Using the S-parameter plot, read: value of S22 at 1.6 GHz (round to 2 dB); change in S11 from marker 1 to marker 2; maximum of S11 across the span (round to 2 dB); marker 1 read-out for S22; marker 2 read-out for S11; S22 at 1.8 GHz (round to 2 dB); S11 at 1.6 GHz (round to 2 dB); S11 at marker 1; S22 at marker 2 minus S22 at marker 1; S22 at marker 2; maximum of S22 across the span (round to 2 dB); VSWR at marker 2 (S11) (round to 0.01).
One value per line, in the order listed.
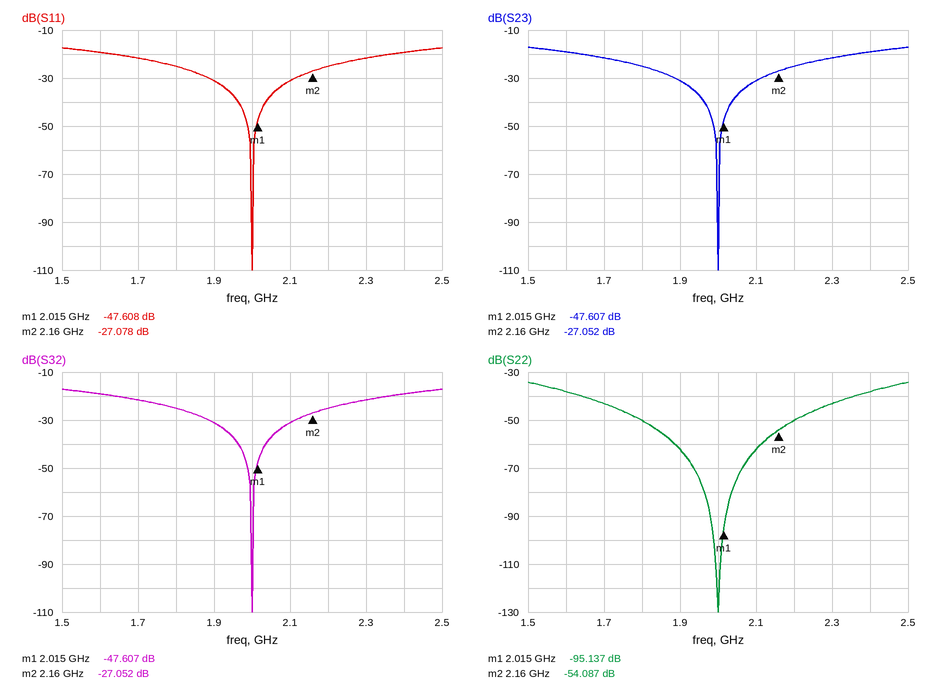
-38 dB
20.530 dB
-18 dB
-95.137 dB
-27.078 dB
-50 dB
-20 dB
-47.608 dB
41.050 dB
-54.087 dB
-34 dB
1.09
